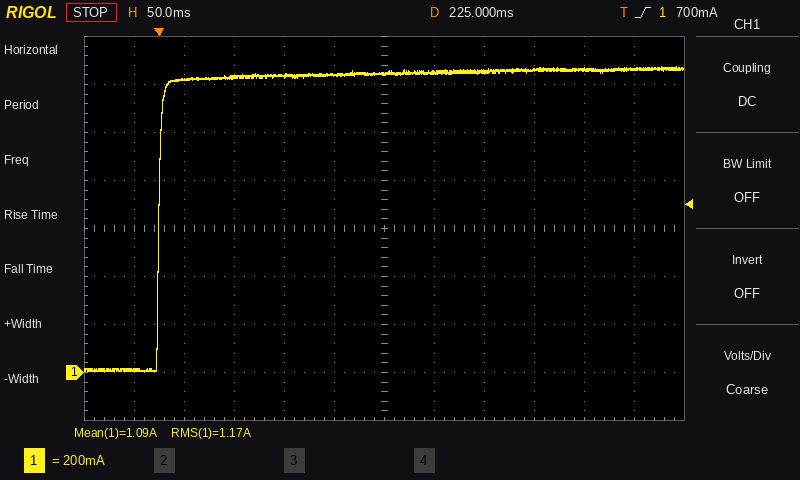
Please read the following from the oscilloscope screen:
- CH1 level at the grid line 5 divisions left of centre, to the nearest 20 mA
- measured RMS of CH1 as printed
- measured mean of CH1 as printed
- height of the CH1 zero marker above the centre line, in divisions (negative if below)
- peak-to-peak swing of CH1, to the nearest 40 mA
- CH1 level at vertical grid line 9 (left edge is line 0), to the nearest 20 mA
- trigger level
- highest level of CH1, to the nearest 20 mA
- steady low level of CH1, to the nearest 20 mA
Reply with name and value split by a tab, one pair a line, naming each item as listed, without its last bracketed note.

CH1 level at the grid line 5 divisions left of centre, to the nearest 20 mA	20 mA
measured RMS of CH1 as printed	1.17 A
measured mean of CH1 as printed	1.09 A
height of the CH1 zero marker above the centre line, in divisions	-3.0 div
peak-to-peak swing of CH1, to the nearest 40 mA	1.28 A
CH1 level at vertical grid line 9 (left edge is line 0), to the nearest 20 mA	1.26 A
trigger level	700 mA
highest level of CH1, to the nearest 20 mA	1.28 A
steady low level of CH1, to the nearest 20 mA	20 mA
